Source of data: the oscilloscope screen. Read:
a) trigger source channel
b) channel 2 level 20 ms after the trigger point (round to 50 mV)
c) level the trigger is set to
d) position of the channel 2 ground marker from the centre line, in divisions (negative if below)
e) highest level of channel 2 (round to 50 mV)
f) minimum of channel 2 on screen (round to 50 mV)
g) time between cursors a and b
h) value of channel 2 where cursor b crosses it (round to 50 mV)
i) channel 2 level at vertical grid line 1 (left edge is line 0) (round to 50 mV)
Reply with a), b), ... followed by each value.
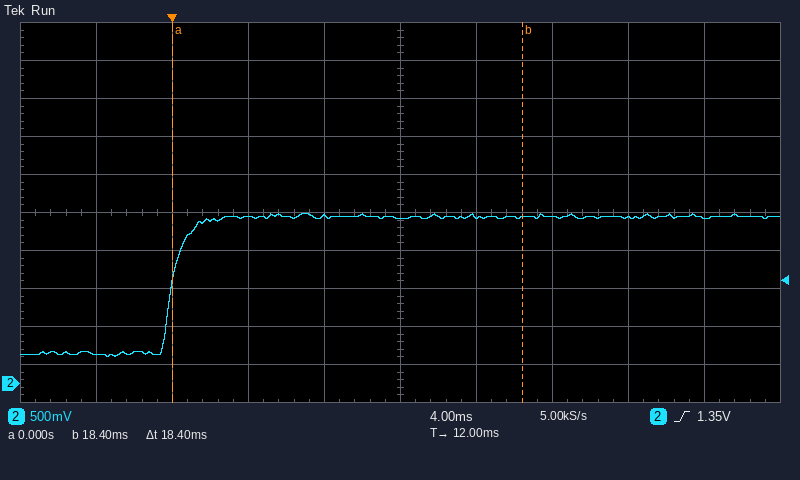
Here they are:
a) channel 2
b) 2.20 V
c) 1.35 V
d) -4.5 div
e) 2.25 V
f) 350 mV
g) 18.4 ms
h) 2.20 V
i) 400 mV
